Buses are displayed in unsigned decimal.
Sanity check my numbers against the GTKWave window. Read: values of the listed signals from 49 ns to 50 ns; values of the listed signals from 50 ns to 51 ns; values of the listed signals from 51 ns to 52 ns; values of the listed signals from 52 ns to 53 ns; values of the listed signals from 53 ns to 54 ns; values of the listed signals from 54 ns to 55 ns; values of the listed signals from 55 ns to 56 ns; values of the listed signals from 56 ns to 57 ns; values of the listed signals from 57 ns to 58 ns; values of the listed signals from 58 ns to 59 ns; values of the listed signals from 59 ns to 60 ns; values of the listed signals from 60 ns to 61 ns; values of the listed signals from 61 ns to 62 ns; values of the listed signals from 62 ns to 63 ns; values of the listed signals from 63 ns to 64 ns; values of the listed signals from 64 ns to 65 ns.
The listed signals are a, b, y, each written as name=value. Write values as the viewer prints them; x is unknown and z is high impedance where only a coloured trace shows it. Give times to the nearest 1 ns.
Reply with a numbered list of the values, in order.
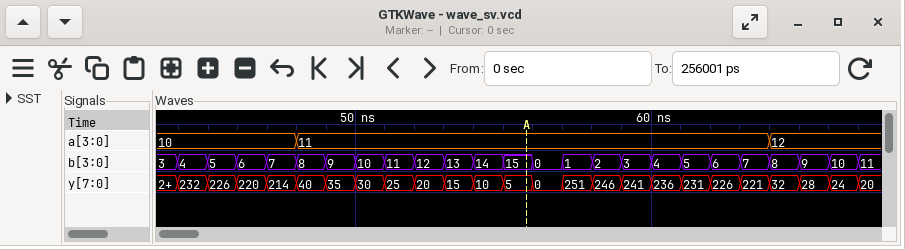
1. a=11, b=9, y=35
2. a=11, b=10, y=30
3. a=11, b=11, y=25
4. a=11, b=12, y=20
5. a=11, b=13, y=15
6. a=11, b=14, y=10
7. a=11, b=15, y=5
8. a=11, b=0, y=0
9. a=11, b=1, y=251
10. a=11, b=2, y=246
11. a=11, b=3, y=241
12. a=11, b=4, y=236
13. a=11, b=5, y=231
14. a=11, b=6, y=226
15. a=11, b=7, y=221
16. a=12, b=8, y=32
